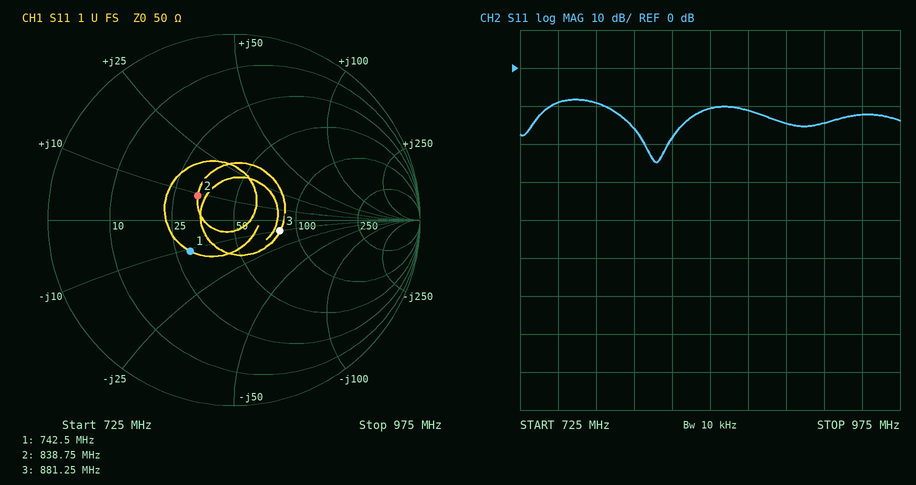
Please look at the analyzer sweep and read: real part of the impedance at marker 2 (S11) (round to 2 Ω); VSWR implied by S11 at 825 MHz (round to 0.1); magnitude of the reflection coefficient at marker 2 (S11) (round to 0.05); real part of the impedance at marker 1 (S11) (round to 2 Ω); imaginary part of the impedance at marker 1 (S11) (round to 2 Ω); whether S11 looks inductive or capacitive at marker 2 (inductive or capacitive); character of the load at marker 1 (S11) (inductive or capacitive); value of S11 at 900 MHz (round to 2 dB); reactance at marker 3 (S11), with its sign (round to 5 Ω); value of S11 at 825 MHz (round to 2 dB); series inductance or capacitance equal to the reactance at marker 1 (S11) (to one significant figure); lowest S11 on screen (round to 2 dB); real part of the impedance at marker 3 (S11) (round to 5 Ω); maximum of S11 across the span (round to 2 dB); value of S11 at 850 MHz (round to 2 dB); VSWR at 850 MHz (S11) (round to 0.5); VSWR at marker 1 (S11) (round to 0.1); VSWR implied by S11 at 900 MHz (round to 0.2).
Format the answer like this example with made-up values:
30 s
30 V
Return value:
32 Ω
1.3
0.25
30 Ω
-10 Ω
inductive
capacitive
-14 dB
-10 Ω
-18 dB
20 pF
-24 dB
80 Ω
-8 dB
-10 dB
2.0
1.8
1.4
